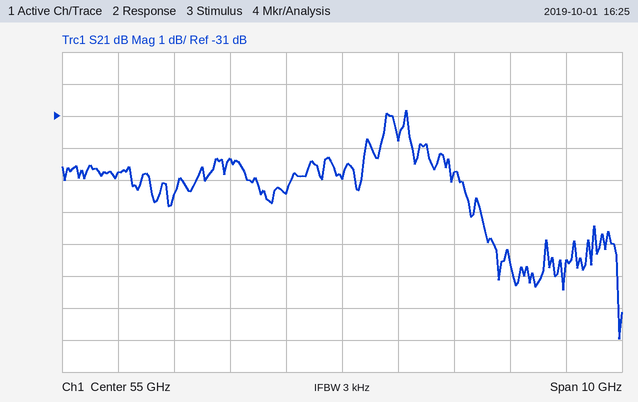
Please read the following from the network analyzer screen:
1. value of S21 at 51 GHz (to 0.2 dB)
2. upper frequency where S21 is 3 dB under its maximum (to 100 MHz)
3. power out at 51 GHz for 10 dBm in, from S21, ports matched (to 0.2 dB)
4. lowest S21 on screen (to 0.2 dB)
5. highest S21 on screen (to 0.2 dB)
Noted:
-32.8 dB
57.3 GHz
-22.8 dBm
-38.0 dB
-30.8 dB
